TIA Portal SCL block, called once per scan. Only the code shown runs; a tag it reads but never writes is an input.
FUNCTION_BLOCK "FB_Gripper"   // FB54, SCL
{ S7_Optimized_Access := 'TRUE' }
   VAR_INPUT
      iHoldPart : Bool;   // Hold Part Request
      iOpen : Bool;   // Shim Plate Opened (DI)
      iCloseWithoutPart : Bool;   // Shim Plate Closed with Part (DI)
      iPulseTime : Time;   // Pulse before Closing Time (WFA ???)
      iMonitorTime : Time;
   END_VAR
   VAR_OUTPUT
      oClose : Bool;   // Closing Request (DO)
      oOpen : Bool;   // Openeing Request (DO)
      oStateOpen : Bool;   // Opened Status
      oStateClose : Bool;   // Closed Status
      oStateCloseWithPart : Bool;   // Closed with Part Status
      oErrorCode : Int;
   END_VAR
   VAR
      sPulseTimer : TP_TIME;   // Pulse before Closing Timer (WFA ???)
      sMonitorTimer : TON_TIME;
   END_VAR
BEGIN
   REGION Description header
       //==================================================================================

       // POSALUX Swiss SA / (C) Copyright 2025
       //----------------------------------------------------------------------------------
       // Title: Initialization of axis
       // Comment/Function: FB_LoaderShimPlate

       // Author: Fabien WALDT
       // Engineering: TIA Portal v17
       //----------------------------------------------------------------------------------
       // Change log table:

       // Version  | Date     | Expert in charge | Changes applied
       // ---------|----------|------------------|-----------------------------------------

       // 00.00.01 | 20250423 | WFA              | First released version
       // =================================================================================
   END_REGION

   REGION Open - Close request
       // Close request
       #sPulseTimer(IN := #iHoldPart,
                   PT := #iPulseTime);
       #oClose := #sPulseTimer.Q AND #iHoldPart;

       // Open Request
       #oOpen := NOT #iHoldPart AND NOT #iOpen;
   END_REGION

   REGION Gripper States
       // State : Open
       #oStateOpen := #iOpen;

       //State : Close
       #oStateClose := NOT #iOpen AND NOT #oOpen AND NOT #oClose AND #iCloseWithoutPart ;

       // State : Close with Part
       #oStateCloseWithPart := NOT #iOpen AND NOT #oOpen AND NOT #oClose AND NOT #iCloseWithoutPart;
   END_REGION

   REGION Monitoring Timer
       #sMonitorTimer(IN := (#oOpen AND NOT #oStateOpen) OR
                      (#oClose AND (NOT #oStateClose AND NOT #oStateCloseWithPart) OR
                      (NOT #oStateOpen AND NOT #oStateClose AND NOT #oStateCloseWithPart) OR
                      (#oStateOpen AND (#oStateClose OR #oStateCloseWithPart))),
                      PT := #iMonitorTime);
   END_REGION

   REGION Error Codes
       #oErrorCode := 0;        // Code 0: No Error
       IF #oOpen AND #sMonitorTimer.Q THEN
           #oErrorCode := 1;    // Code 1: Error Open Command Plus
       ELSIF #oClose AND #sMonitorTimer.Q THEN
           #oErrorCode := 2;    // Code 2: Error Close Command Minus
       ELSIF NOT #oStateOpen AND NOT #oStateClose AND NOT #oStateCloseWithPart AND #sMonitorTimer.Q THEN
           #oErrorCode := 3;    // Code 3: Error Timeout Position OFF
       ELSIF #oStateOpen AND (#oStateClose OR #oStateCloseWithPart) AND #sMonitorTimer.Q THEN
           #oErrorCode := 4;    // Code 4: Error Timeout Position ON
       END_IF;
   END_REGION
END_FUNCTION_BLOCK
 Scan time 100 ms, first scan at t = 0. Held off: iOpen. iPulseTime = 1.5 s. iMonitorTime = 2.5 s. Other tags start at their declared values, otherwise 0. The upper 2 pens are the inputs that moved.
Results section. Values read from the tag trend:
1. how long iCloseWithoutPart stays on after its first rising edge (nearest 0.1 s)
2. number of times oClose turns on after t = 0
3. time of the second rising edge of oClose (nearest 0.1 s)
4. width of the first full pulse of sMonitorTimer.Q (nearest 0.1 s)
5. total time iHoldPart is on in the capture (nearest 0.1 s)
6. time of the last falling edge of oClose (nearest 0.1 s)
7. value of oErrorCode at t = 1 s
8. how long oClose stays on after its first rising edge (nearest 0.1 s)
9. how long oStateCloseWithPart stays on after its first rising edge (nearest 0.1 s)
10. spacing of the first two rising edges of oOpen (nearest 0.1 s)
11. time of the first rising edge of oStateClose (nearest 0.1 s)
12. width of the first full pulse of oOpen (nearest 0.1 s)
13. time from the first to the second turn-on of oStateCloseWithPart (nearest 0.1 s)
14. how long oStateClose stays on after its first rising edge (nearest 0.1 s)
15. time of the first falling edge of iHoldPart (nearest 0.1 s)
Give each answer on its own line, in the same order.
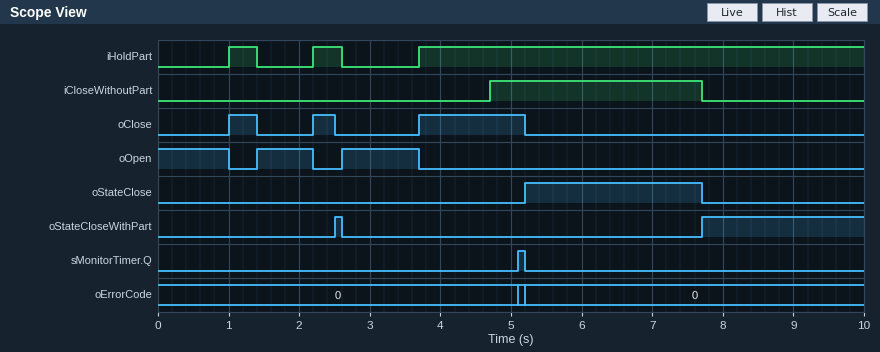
3.0 s
3
2.2 s
0.1 s
7.1 s
5.2 s
0
0.4 s
0.1 s
1.2 s
5.2 s
0.8 s
5.2 s
2.5 s
1.4 s
